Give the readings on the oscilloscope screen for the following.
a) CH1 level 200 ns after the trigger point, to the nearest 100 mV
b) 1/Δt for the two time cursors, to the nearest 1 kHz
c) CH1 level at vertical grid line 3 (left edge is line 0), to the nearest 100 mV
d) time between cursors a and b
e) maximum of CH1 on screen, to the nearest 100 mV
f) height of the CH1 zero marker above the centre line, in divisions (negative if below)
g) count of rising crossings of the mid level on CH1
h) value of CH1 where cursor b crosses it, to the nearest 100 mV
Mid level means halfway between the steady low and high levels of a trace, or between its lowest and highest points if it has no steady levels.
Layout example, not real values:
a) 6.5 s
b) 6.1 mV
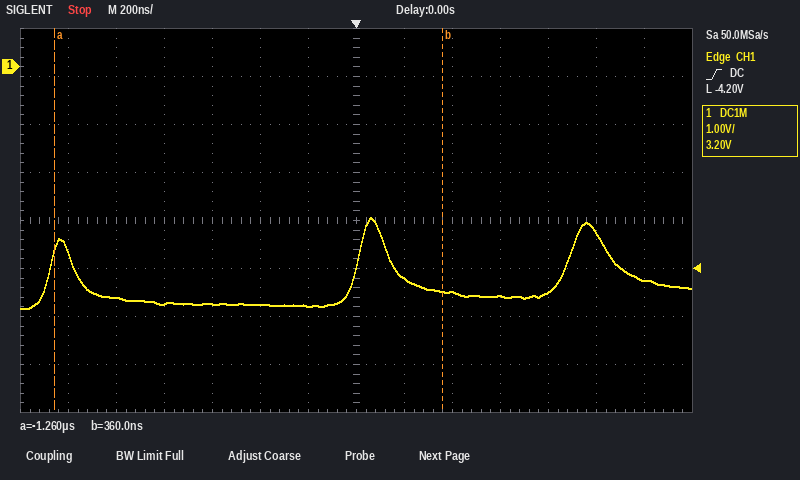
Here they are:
a) -4.4 V
b) 617 kHz
c) -4.9 V
d) 1.62 µs
e) -3.1 V
f) +3.2 div
g) 3
h) -4.7 V
